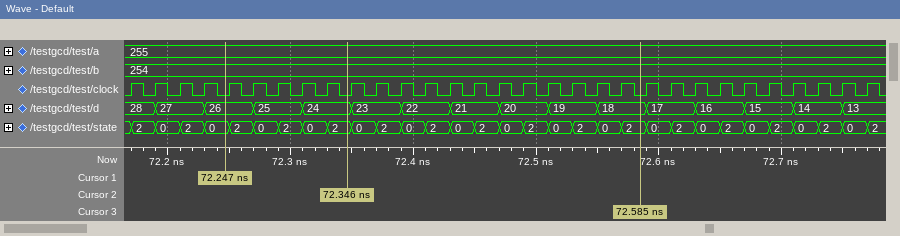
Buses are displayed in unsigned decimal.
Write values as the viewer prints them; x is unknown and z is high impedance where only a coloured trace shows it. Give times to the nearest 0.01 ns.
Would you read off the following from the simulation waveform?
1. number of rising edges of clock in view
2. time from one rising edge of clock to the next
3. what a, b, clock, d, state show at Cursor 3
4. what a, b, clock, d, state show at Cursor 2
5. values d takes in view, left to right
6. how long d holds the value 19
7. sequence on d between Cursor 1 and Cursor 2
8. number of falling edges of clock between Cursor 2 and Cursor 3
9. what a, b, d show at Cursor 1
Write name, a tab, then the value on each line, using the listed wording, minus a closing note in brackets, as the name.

number of rising edges of clock in view	31
time from one rising edge of clock to the next	0.02 ns
what a, b, clock, d, state show at Cursor 3	a=255, b=254, clock=0, d=18, state=2
what a, b, clock, d, state show at Cursor 2	a=255, b=254, clock=0, d=24, state=2
values d takes in view, left to right	28, 27, 26, 25, 24, 23, 22, 21, 20, 19, 18, 17, 16, 15, 14, 13
how long d holds the value 19	0.04 ns
sequence on d between Cursor 1 and Cursor 2	26, 25, 24
number of falling edges of clock between Cursor 2 and Cursor 3	12
what a, b, d show at Cursor 1	a=255, b=254, d=26
